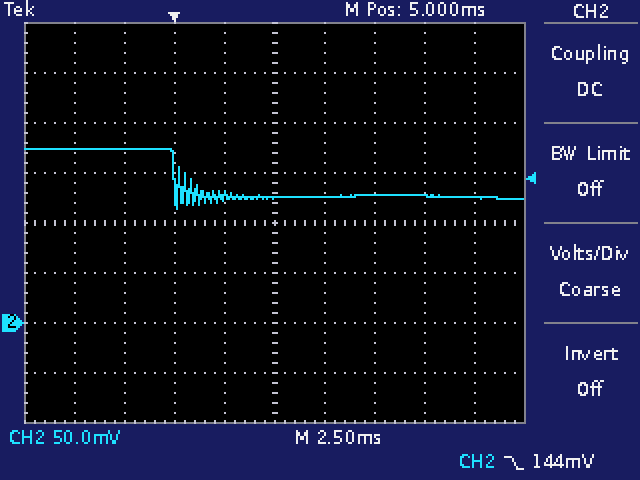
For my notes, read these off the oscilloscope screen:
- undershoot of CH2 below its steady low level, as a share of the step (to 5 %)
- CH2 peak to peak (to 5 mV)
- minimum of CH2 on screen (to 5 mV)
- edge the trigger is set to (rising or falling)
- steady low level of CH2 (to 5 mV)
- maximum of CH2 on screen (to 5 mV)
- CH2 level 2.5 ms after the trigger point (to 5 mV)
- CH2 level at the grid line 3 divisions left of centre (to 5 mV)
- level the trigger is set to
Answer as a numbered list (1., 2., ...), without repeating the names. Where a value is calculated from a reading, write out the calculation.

1. 25 %
2. 175 mV − (115 mV) = 60 mV
3. 115 mV
4. falling
5. 125 mV
6. 175 mV
7. 125 mV
8. 175 mV
9. 144 mV
